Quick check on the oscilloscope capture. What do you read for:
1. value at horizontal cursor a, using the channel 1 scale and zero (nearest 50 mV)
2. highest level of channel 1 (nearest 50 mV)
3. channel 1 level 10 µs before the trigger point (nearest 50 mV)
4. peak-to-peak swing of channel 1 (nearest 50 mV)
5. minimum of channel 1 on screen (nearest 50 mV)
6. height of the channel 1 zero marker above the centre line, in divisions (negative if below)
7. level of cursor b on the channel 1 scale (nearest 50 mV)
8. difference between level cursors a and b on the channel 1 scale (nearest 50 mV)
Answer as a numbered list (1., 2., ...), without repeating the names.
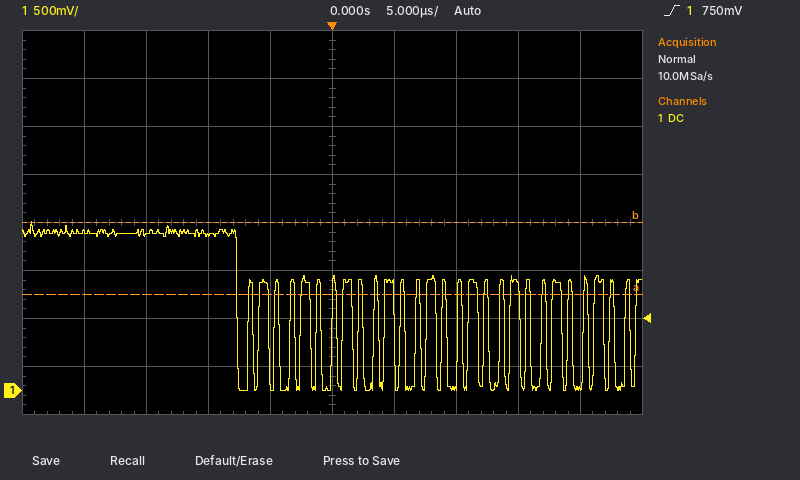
1. 1.00 V
2. 1.75 V
3. 1.60 V
4. 1.75 V
5. 0 mV
6. -3.5 div
7. 1.75 V
8. 750 mV
